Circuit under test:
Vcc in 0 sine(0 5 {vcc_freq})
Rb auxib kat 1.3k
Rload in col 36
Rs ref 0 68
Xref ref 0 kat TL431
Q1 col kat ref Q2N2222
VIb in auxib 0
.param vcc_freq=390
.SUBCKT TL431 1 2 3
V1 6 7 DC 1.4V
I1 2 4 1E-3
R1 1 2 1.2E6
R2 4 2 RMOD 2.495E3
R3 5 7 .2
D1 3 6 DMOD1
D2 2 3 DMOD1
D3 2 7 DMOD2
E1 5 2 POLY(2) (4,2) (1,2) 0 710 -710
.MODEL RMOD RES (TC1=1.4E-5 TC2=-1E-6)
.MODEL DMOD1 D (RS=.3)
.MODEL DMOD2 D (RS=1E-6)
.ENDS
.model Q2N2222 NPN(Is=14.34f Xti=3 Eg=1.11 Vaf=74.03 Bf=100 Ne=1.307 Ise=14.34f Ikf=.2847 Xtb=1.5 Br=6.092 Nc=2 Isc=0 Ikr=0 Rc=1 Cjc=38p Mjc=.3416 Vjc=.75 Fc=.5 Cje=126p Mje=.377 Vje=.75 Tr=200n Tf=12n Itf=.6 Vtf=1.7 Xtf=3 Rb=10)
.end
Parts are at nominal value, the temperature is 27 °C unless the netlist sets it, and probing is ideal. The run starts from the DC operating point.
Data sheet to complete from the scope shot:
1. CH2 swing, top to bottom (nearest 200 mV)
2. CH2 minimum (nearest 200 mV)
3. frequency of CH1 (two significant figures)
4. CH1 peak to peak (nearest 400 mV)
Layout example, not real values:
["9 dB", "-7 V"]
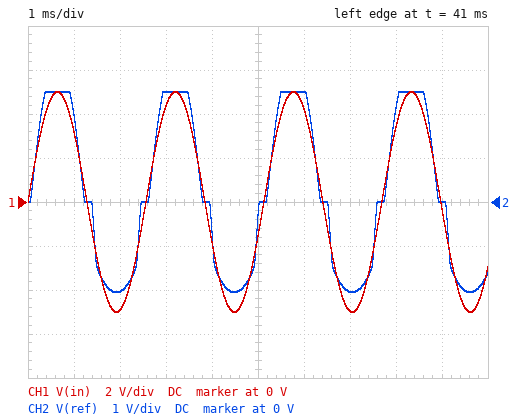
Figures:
["4.6 V", "-2.0 V", "390 Hz", "10.0 V"]
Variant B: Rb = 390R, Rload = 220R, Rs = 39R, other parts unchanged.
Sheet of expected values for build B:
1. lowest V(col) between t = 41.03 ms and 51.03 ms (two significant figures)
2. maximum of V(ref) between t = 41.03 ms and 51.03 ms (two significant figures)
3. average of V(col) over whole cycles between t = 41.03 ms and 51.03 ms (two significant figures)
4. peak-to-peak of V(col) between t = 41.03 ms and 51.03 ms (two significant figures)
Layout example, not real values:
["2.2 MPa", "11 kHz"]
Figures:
["-1.5 V", "1.0 V", "-310 mV", "2.5 V"]
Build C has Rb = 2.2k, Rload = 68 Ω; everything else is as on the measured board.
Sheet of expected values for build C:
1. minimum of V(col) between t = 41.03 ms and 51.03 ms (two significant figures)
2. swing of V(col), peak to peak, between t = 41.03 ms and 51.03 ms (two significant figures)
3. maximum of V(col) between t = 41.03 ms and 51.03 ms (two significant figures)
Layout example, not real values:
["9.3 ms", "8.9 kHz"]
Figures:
["-1.8 V", "4.4 V", "2.6 V"]
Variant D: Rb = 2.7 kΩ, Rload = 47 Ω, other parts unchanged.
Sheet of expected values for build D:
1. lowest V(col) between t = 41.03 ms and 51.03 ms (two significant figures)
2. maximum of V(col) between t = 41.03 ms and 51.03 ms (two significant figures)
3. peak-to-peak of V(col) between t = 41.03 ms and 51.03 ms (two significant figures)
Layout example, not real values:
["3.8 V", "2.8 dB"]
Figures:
["-2.0 V", "3.3 V", "5.3 V"]
